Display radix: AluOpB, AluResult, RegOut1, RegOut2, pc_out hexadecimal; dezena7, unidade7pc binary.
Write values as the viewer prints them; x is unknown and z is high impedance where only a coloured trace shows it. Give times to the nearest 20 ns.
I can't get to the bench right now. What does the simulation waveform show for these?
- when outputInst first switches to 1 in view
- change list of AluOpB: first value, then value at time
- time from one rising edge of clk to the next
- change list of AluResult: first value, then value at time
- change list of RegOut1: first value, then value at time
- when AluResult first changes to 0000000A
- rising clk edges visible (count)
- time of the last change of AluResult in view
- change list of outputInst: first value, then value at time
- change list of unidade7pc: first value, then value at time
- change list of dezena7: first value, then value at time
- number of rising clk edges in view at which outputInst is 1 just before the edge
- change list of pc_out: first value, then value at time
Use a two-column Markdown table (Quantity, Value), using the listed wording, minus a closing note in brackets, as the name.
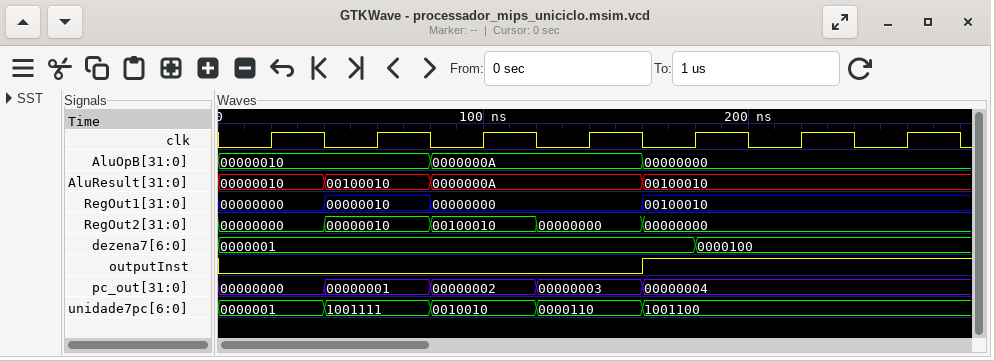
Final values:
| Quantity | Value |
|---|---|
| when outputInst first switches to 1 in view | 160 ns |
| change list of AluOpB: first value, then value at time | 00000010, 0000000A at 80 ns, 00000000 at 160 ns |
| time from one rising edge of clk to the next | 40 ns |
| change list of AluResult: first value, then value at time | 00000010, 00100010 at 40 ns, 0000000A at 80 ns, 00100010 at 160 ns |
| change list of RegOut1: first value, then value at time | 00000000, 00000010 at 40 ns, 00000000 at 80 ns, 00100010 at 160 ns |
| when AluResult first changes to 0000000A | 80 ns |
| rising clk edges visible | 7 |
| time of the last change of AluResult in view | 160 ns |
| change list of outputInst: first value, then value at time | 0, 1 at 160 ns |
| change list of unidade7pc: first value, then value at time | 0000001, 1001111 at 40 ns, 0010010 at 80 ns, 0000110 at 120 ns, 1001100 at 160 ns |
| change list of dezena7: first value, then value at time | 0000001, 0000100 at 180 ns |
| number of rising clk edges in view at which outputInst is 1 just before the edge | 3 |
| change list of pc_out: first value, then value at time | 00000000, 00000001 at 40 ns, 00000002 at 80 ns, 00000003 at 120 ns, 00000004 at 160 ns |
